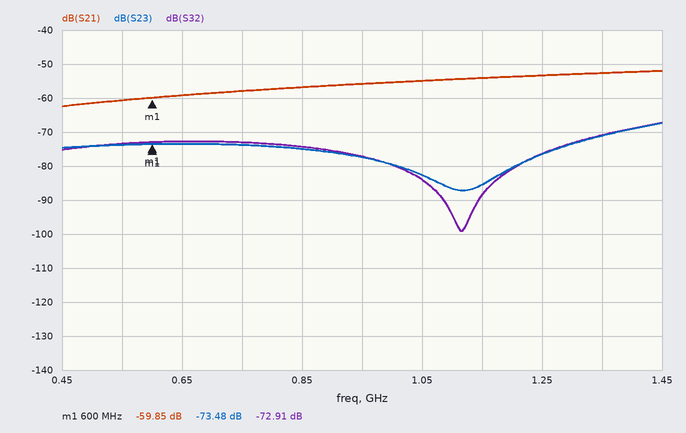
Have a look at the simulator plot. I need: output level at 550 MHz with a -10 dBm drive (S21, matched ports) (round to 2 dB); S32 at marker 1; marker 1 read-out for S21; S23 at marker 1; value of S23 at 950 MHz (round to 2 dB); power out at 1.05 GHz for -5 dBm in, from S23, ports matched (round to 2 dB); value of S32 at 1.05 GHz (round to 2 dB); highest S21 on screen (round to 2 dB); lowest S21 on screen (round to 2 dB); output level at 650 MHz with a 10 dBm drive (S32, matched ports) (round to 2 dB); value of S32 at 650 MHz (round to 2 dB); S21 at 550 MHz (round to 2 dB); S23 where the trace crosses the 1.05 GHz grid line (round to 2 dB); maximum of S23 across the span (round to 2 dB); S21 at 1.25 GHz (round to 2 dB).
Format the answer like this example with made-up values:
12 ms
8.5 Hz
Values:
-70 dBm
-72.91 dB
-59.85 dB
-73.48 dB
-78 dB
-88 dBm
-84 dB
-52 dB
-62 dB
-62 dBm
-72 dB
-60 dB
-82 dB
-68 dB
-54 dB
